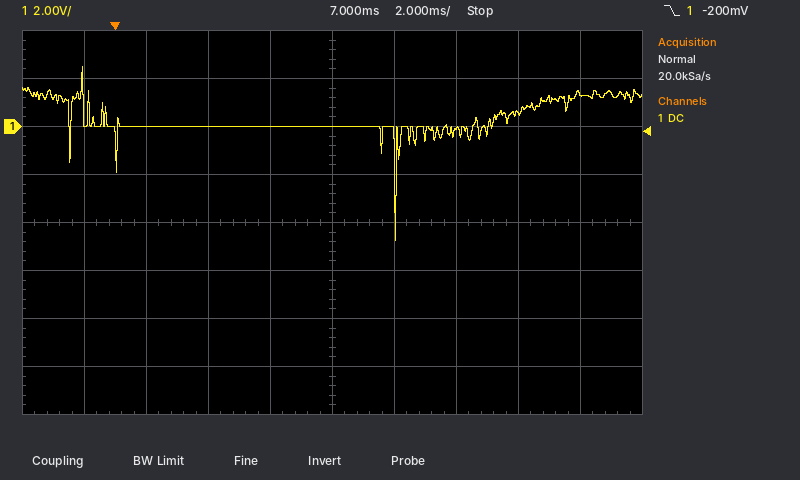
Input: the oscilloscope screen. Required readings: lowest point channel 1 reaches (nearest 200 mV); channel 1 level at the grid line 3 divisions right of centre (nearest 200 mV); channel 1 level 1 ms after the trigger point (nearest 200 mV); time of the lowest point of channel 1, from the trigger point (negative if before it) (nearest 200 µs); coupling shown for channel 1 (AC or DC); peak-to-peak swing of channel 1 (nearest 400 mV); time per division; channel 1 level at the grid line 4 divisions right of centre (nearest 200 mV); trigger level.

-4.8 V
600 mV
0.0 V
+9.0 ms
DC
7.2 V
2 ms
1.4 V
-200 mV
